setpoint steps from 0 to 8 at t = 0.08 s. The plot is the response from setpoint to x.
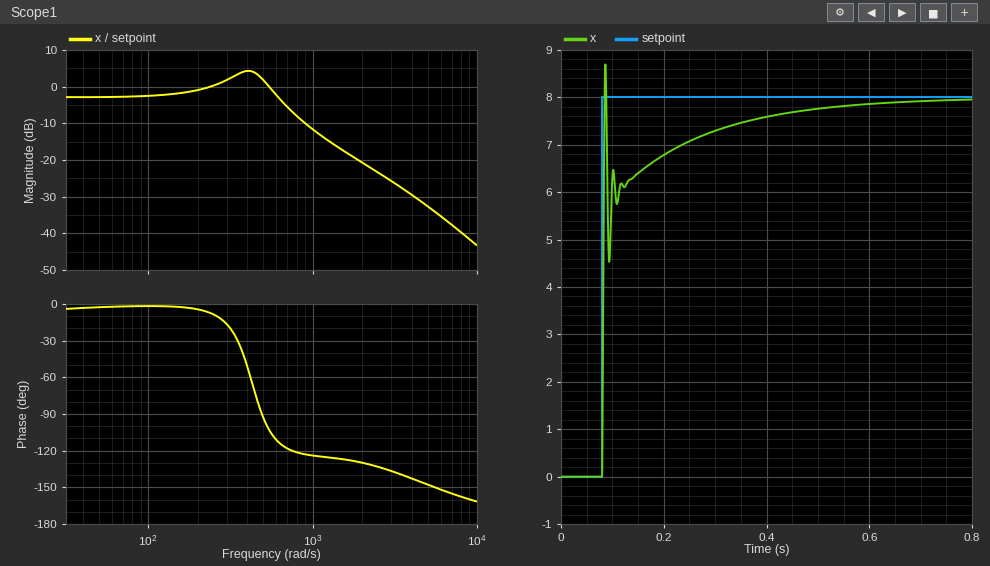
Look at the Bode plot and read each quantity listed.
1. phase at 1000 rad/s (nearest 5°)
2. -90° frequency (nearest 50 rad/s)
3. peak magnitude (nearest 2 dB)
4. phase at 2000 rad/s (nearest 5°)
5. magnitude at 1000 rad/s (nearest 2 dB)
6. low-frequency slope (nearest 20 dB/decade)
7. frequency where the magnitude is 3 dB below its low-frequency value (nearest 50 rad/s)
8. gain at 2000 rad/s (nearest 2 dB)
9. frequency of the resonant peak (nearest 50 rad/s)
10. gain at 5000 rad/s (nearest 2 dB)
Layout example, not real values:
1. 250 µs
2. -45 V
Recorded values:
1. -125°
2. 500 rad/s
3. 4 dB
4. -130°
5. -12 dB
6. 0 dB/decade
7. 700 rad/s
8. -20 dB
9. 400 rad/s
10. -32 dB
